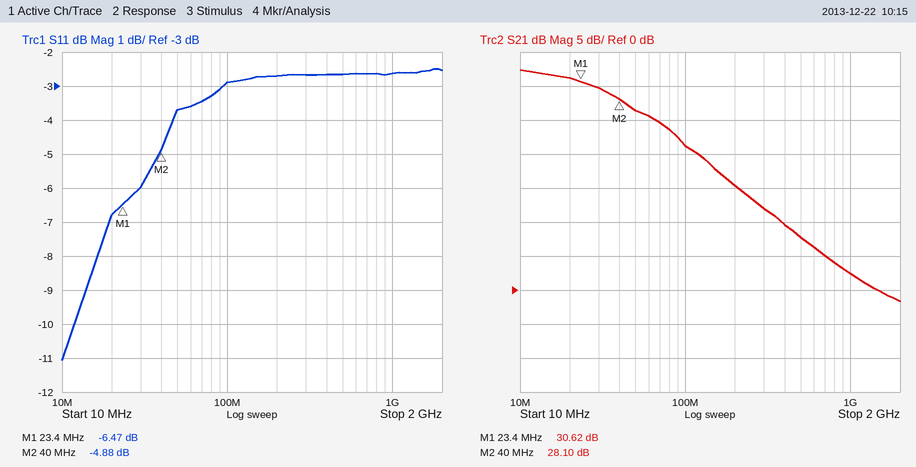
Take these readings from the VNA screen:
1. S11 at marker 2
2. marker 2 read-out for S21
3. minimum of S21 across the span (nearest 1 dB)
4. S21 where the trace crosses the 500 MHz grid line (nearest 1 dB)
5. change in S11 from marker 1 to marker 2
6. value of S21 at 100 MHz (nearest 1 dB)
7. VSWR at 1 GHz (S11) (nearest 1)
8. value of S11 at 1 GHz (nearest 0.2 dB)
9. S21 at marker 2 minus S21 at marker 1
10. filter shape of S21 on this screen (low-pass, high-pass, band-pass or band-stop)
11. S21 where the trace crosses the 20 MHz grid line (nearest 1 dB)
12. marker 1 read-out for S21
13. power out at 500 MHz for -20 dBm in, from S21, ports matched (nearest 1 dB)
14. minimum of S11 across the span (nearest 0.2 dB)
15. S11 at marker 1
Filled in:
-4.88 dB
28.10 dB
-2 dB
8 dB
1.59 dB
21 dB
7
-2.6 dB
-2.52 dB
low-pass
31 dB
30.62 dB
-12 dBm
-11.0 dB
-6.47 dB
